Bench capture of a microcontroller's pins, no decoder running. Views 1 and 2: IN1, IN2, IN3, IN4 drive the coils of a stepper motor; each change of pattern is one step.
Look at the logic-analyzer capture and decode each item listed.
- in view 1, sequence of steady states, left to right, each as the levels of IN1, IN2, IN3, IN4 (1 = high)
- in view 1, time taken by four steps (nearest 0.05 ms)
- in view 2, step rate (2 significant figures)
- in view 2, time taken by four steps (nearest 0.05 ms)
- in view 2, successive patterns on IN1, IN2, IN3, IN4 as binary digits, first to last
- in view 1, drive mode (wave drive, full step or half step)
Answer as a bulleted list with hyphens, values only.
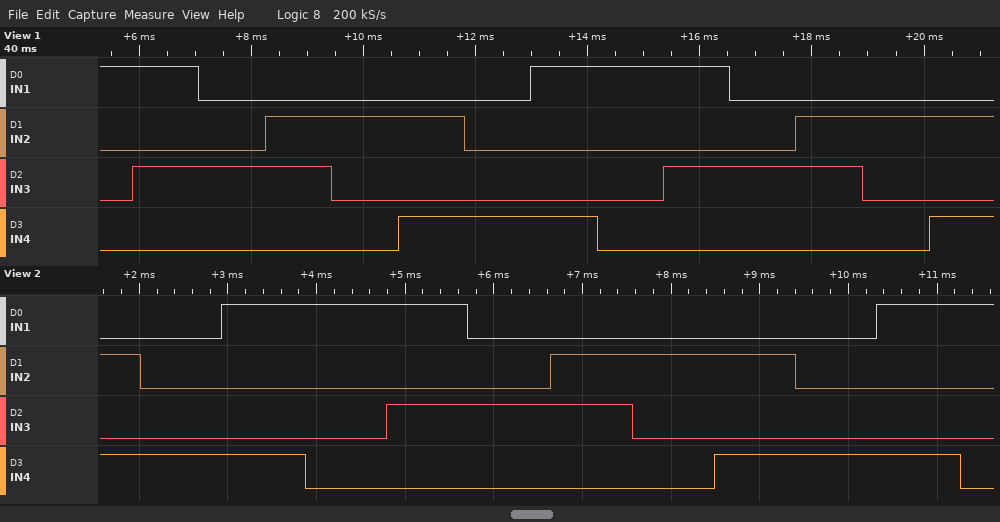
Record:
- 1000 1010 0010 0110 0100 0101 0001 1001 1000 1010 0010 0110 0100 0101
- 4.75 ms
- 1100 steps/s
- 3.70 ms
- 0101 0001 1001 1000 1010 0010 0110 0100 0101 0001 1001 1000
- half step
